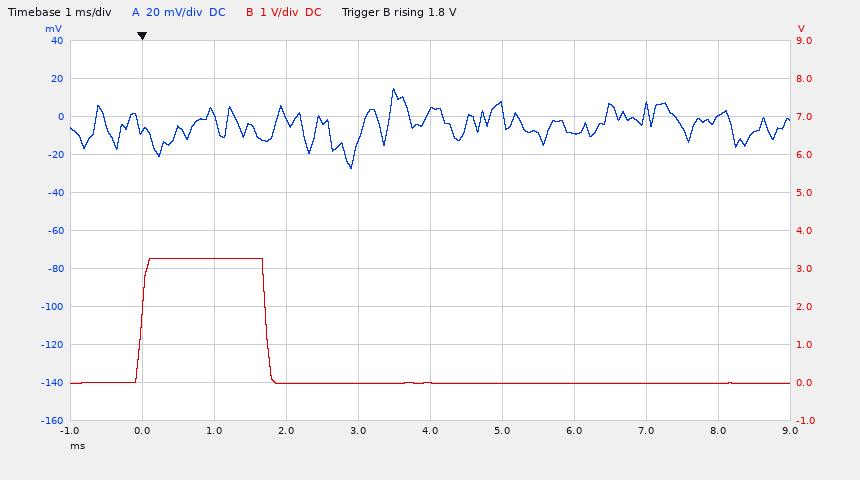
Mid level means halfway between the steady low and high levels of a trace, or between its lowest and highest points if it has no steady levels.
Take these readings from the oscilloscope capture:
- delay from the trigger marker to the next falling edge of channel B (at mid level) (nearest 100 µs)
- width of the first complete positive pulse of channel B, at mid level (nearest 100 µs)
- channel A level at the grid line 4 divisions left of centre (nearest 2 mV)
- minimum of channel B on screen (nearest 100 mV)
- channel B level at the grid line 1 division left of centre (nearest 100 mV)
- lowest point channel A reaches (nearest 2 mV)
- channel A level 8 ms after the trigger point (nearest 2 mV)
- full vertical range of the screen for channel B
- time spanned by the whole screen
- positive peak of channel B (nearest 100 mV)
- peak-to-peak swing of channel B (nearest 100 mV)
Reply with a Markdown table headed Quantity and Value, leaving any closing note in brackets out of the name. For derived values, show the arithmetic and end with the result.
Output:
| Quantity | Value |
|---|---|
| delay from the trigger marker to the next falling edge of channel B (at mid level) | 1.7 ms |
| width of the first complete positive pulse of channel B, at mid level | 1.7 ms |
| channel A level at the grid line 4 divisions left of centre | -8 mV |
| minimum of channel B on screen | 0.0 V |
| channel B level at the grid line 1 division left of centre | 0.0 V |
| lowest point channel A reaches | -28 mV |
| channel A level 8 ms after the trigger point | 0 mV |
| full vertical range of the screen for channel B | 10 V |
| time spanned by the whole screen | 10 ms |
| positive peak of channel B | 3.3 V |
| peak-to-peak swing of channel B | 3.3 V − (0.0 V) = 3.3 V |
